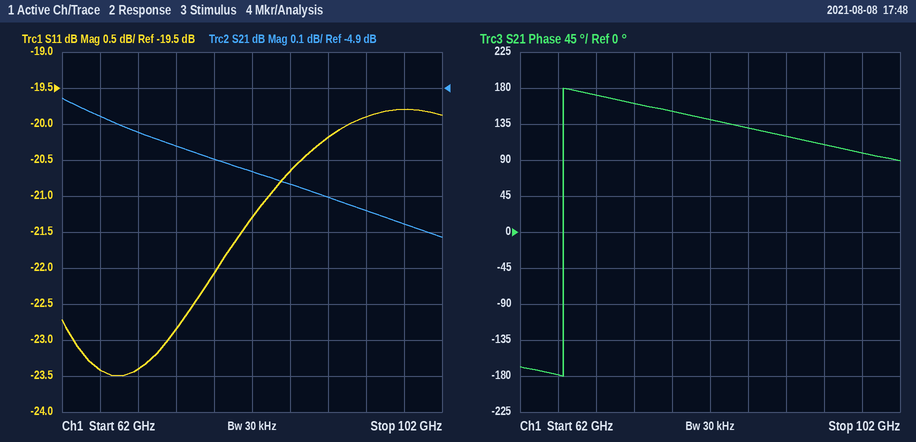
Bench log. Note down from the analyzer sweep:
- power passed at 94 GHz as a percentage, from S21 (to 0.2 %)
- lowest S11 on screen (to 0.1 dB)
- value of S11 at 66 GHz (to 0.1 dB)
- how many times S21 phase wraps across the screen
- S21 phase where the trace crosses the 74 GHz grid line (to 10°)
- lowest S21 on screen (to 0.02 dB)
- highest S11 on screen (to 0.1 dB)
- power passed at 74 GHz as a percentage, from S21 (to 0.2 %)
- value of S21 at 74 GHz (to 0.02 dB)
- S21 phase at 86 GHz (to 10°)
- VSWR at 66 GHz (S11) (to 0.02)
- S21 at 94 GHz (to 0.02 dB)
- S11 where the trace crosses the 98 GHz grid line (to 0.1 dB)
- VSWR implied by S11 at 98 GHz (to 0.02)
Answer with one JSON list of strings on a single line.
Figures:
["30.0 %", "-23.5 dB", "-23.4 dB", "1", "160°", "-5.32 dB", "-19.8 dB", "31.2 %", "-5.06 dB", "130°", "1.14", "-5.24 dB", "-19.8 dB", "1.22"]
